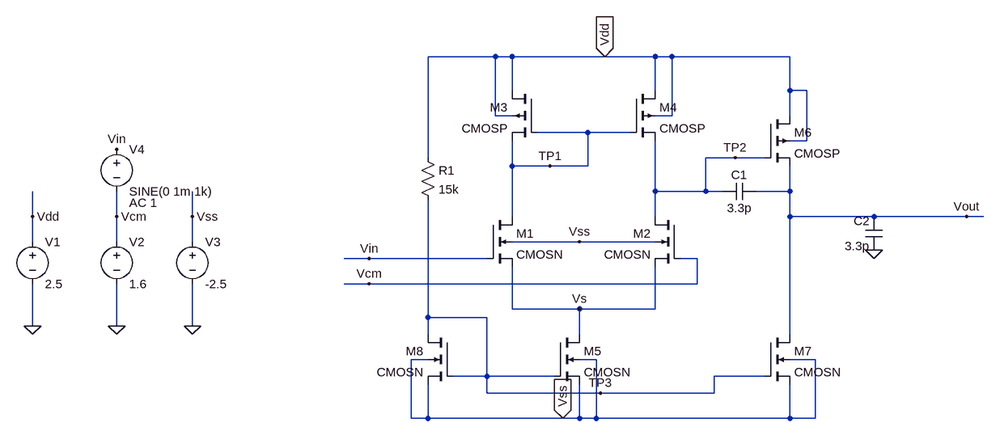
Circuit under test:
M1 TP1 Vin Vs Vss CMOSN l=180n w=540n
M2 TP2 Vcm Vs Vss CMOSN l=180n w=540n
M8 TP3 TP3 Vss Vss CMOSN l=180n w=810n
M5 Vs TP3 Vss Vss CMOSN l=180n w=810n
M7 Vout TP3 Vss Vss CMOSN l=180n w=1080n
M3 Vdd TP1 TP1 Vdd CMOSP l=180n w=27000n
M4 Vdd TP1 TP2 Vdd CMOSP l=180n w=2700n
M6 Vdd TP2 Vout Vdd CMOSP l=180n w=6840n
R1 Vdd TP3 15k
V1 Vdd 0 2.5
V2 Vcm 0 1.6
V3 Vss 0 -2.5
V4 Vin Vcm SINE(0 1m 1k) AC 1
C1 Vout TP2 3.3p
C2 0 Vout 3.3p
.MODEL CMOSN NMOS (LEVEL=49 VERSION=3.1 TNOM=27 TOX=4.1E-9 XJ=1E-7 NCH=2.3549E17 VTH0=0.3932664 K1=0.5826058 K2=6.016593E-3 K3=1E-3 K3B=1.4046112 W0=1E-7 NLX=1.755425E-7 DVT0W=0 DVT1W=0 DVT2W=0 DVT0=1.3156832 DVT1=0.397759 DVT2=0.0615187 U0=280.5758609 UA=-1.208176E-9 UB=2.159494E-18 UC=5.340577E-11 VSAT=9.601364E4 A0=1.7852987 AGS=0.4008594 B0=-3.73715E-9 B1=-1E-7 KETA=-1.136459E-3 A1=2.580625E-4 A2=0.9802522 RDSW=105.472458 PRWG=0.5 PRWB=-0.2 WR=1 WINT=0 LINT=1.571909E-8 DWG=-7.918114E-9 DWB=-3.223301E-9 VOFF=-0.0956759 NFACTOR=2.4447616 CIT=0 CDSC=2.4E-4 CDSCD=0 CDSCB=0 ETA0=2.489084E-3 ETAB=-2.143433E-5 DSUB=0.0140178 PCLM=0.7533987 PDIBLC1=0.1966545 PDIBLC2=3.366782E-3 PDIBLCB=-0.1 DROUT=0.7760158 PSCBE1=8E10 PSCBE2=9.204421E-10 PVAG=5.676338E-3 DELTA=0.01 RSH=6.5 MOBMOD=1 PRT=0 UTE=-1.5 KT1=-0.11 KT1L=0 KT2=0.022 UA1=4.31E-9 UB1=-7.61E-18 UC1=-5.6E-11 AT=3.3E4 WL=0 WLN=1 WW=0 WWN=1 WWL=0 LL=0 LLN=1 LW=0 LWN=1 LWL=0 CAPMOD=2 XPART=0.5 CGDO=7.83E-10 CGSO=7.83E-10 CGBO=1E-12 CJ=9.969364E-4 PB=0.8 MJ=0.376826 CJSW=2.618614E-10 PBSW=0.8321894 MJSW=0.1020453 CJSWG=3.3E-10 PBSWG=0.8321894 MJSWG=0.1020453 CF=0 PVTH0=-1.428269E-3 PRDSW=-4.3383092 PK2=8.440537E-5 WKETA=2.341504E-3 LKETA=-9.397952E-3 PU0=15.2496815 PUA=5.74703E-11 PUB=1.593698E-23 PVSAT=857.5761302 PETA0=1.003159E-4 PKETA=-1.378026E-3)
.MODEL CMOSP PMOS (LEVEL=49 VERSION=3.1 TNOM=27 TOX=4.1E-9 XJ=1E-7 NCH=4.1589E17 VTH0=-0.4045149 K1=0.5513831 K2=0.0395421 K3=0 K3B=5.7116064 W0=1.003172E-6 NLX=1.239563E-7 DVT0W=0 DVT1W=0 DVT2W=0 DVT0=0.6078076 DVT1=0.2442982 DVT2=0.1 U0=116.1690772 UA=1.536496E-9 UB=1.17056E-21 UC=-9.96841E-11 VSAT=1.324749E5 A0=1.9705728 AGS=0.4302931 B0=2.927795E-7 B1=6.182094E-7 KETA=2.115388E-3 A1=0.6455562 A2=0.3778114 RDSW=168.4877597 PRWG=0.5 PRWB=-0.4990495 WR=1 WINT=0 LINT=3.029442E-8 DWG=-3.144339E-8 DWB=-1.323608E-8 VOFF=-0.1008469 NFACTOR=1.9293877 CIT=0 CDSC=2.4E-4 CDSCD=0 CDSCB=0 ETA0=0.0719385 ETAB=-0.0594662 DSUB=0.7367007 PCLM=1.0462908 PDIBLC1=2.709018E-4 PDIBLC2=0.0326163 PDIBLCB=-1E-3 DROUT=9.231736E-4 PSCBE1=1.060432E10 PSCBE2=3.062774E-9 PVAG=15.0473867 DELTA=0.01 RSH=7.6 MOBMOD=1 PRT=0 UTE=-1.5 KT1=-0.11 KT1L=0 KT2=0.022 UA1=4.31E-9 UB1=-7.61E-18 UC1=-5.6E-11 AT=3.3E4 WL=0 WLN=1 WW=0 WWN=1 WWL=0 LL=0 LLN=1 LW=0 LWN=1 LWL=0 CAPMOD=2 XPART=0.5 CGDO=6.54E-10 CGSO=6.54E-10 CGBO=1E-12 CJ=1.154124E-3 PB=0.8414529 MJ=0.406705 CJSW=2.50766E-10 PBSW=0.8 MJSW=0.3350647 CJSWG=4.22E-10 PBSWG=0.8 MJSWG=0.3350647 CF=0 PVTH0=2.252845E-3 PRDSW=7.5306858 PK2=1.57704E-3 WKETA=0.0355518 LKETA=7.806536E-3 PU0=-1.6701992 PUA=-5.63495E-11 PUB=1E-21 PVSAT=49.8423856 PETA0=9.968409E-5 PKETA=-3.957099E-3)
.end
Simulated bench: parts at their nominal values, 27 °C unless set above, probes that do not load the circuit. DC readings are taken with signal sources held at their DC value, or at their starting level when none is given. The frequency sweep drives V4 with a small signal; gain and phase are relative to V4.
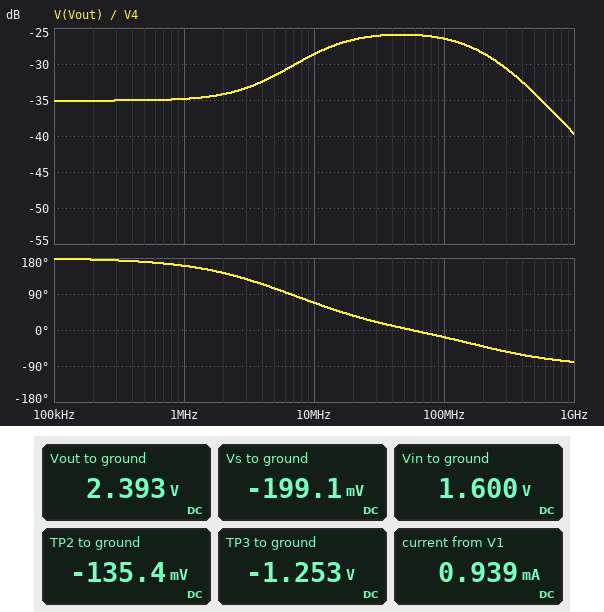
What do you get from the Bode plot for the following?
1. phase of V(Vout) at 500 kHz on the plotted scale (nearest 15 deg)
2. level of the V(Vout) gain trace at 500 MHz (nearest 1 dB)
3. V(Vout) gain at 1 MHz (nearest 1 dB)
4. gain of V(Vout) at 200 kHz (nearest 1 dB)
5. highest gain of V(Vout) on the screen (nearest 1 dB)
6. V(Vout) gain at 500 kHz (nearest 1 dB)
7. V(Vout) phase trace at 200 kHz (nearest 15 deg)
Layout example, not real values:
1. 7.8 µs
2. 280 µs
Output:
1. 165 deg
2. -34 dB
3. -35 dB
4. -35 dB
5. -26 dB
6. -35 dB
7. 180 deg
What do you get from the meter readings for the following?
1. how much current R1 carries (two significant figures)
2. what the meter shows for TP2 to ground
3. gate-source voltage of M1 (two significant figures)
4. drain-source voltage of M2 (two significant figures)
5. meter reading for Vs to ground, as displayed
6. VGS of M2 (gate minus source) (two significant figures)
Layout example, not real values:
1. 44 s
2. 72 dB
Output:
1. 250 µA
2. -135.4 mV
3. 1.8 V
4. 64 mV
5. -199.1 mV
6. 1.8 V
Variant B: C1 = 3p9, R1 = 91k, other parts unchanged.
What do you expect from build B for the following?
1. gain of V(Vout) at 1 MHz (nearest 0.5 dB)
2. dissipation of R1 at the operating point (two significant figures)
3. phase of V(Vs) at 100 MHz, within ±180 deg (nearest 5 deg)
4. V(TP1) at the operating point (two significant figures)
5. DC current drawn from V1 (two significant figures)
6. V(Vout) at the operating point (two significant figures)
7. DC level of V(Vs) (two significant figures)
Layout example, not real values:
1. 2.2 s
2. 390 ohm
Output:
1. -38.5 dB
2. 200 µW
3. -5 deg
4. 1.9 V
5. 240 µA
6. 2.5 V
7. 280 mV
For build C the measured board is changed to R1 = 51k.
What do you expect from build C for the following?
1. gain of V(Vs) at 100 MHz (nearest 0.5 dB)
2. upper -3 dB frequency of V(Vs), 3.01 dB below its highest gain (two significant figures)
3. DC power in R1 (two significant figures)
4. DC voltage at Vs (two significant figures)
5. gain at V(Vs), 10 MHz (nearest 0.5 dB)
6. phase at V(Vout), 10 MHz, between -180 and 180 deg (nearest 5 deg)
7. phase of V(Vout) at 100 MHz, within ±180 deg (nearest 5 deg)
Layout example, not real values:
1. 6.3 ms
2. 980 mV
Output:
1. -7.5 dB
2. 12 MHz
3. 340 µW
4. 180 mV
5. -4.5 dB
6. 50 deg
7. -25 deg
